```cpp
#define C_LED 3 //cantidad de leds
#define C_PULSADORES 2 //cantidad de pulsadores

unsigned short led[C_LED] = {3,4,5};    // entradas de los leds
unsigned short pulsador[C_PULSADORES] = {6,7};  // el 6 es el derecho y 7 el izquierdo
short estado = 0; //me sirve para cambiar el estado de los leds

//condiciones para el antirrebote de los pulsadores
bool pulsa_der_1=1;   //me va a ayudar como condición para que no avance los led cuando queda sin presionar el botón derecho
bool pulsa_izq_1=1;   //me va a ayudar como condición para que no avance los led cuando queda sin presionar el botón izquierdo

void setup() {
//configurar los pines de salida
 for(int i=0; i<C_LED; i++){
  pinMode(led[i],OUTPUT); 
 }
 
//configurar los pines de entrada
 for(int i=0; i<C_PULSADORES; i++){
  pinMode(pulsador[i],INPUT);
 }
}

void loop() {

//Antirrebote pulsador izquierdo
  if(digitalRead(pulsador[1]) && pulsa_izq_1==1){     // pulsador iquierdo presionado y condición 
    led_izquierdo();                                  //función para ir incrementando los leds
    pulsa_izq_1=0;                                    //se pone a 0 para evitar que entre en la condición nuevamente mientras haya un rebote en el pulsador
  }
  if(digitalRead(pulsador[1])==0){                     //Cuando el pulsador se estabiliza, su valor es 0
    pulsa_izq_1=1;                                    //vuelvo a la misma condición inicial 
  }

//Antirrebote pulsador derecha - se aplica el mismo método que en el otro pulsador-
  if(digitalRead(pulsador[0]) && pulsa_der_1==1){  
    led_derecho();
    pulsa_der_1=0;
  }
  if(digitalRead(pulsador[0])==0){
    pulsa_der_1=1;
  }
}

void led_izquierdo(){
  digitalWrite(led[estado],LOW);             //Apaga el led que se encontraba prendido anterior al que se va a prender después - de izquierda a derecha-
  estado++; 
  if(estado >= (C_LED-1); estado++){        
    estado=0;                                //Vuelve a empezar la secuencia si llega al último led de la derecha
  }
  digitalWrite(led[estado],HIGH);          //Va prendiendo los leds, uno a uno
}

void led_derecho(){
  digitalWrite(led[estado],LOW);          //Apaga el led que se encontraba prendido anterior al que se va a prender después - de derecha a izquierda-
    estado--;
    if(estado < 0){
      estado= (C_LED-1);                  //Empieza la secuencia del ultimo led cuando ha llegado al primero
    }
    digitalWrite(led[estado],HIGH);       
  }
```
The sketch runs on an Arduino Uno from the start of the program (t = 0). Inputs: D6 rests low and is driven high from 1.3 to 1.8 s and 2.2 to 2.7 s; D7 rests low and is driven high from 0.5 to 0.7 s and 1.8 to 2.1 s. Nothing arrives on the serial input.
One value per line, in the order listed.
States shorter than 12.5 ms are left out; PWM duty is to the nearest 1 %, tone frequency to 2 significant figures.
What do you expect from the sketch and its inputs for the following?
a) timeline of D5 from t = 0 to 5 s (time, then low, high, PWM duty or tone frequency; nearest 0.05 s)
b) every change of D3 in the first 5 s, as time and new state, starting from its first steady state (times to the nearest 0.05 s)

0 s low; 1.3 s high; 1.8 s low; 2.2 s high
0 s low; 0.5 s high; 1.3 s low; 1.8 s high; 2.2 s low
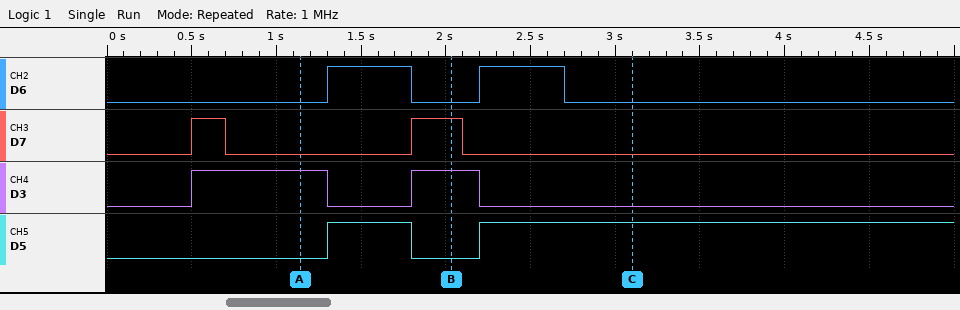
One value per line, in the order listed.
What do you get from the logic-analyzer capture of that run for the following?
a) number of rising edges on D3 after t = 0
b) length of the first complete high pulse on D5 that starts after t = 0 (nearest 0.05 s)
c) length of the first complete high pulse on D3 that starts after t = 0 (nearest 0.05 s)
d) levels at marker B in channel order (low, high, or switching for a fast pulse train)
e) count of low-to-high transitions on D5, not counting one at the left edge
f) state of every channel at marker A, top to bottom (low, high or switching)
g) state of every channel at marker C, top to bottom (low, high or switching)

2
0.50 s
0.80 s
D6 low, D7 high, D3 high, D5 low
2
D6 low, D7 low, D3 high, D5 low
D6 low, D7 low, D3 low, D5 high
